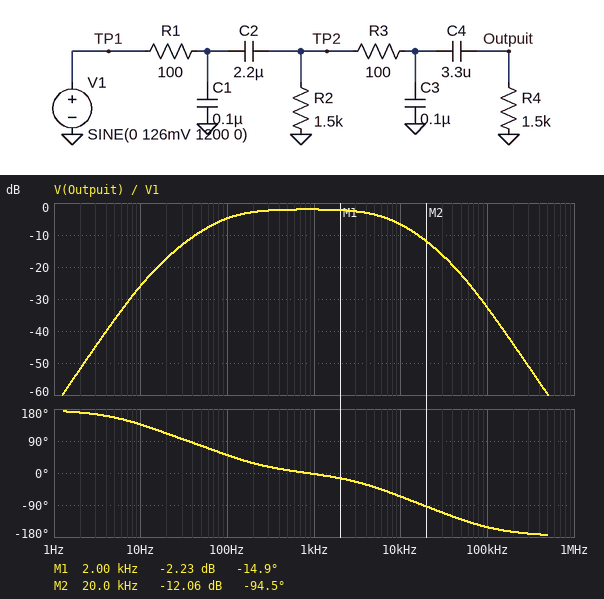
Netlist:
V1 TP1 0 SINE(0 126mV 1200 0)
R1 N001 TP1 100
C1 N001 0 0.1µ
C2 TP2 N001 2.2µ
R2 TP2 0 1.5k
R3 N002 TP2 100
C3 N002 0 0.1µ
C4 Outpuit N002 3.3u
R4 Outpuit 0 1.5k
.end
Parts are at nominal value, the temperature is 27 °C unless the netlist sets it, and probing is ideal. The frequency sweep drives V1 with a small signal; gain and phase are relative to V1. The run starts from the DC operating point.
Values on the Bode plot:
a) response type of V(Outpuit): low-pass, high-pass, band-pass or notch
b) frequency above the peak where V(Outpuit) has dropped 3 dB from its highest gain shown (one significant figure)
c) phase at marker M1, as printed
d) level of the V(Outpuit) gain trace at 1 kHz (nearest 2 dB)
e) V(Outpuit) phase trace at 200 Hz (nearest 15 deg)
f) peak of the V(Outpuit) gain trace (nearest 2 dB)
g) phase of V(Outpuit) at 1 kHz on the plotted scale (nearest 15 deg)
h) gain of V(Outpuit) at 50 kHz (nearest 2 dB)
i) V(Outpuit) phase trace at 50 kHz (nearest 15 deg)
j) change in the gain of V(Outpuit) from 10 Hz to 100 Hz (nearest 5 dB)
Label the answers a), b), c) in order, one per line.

a) band-pass
b) 7 kHz
c) -14.9 deg
d) -2 dB
e) 30 deg
f) -2 dB
g) 0 deg
h) -22 dB
i) -135 deg
j) 20 dB
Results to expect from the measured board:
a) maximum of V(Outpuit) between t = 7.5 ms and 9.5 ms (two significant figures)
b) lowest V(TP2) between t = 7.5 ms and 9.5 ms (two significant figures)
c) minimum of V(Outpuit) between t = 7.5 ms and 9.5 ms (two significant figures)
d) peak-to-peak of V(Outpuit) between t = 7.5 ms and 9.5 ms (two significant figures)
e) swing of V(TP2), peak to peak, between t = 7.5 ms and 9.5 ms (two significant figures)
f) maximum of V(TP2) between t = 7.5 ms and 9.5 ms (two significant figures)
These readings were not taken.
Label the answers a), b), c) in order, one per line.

a) 100 mV
b) -110 mV
c) -100 mV
d) 200 mV
e) 210 mV
f) 110 mV
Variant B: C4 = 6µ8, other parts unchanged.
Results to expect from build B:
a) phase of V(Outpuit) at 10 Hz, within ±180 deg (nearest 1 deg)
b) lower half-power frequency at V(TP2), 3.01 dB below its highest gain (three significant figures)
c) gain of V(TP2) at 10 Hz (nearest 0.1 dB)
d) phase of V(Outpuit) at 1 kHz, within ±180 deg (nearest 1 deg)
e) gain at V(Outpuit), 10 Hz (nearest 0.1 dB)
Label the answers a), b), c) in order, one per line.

a) 118 deg
b) 83.4 Hz
c) -16.9 dB
d) -4 deg
e) -22.5 dB
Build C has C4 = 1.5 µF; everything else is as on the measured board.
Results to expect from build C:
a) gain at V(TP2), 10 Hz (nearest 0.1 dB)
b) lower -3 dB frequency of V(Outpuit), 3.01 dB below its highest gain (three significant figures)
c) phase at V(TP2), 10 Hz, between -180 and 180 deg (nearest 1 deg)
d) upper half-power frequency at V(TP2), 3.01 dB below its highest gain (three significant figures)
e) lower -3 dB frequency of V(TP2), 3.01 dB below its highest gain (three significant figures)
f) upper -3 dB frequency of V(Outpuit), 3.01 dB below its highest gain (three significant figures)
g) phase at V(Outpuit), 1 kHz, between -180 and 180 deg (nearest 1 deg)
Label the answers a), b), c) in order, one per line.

a) -14.4 dB
b) 121 Hz
c) 70 deg
d) 8.97 kHz
e) 82.3 Hz
f) 7.32 kHz
g) -1 deg
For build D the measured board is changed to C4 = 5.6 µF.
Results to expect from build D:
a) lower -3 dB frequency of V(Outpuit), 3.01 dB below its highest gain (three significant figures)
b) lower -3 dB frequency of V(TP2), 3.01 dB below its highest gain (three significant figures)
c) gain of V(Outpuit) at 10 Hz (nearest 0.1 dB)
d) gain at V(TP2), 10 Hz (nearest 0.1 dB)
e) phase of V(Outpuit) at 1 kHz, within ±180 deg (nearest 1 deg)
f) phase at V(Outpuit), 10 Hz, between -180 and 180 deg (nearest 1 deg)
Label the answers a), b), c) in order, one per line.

a) 87.4 Hz
b) 84.1 Hz
c) -23.2 dB
d) -16.4 dB
e) -4 deg
f) 123 deg
